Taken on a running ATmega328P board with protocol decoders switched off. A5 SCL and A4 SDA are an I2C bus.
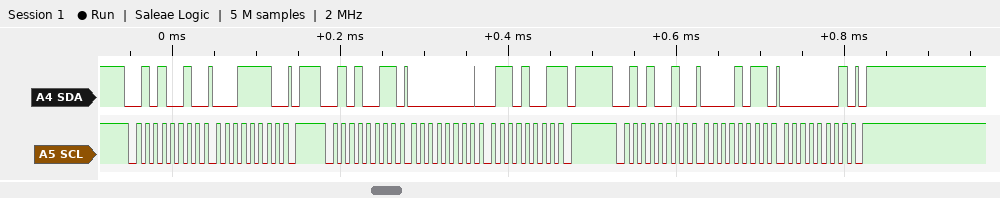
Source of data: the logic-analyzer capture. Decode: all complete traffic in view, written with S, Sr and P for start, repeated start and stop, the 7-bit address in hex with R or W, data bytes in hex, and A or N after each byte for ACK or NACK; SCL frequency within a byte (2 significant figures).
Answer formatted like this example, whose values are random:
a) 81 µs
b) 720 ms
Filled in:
a) S 29W A 1E A P S 29R A 00 A 69 N P S 29W A 0B A 01 A P
b) 100 kHz
